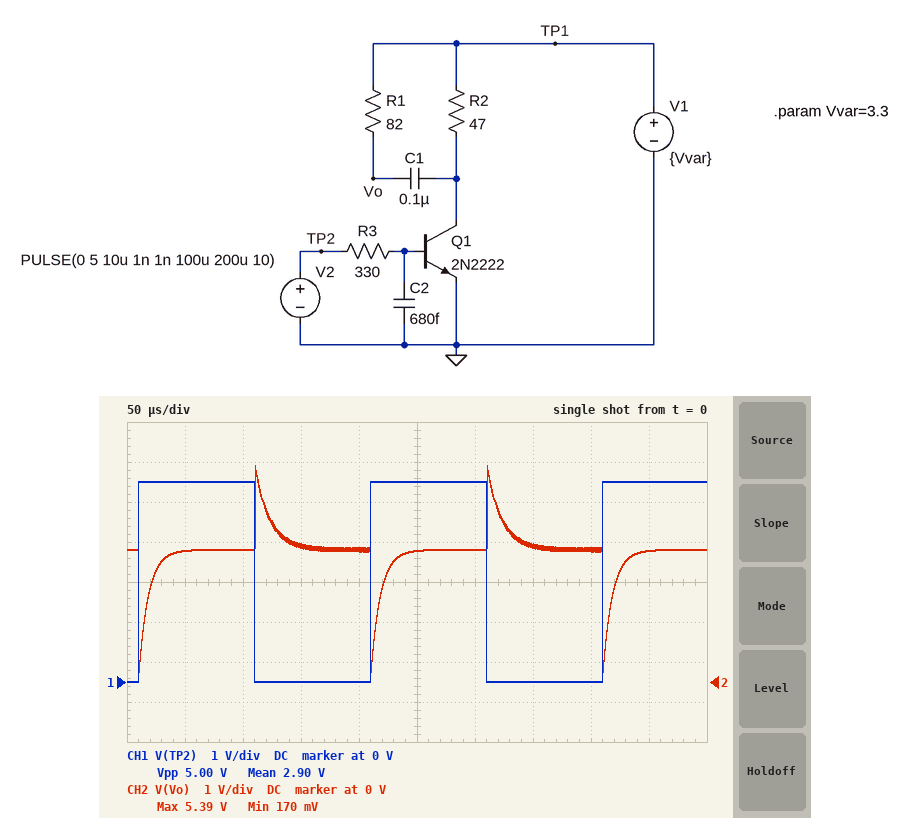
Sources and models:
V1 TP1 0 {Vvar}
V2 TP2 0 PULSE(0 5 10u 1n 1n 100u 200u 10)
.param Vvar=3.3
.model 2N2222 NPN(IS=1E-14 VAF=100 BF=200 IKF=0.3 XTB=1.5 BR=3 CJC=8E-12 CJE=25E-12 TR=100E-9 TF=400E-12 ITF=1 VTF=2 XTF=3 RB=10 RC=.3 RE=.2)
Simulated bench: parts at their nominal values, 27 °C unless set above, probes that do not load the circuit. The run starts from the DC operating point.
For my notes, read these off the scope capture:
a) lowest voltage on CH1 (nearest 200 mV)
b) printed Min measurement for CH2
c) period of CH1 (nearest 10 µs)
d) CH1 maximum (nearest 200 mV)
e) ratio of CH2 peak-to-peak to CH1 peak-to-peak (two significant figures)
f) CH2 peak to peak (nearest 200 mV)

0 V
170 mV
200 µs
5.0 V
1.0
5.2 V
